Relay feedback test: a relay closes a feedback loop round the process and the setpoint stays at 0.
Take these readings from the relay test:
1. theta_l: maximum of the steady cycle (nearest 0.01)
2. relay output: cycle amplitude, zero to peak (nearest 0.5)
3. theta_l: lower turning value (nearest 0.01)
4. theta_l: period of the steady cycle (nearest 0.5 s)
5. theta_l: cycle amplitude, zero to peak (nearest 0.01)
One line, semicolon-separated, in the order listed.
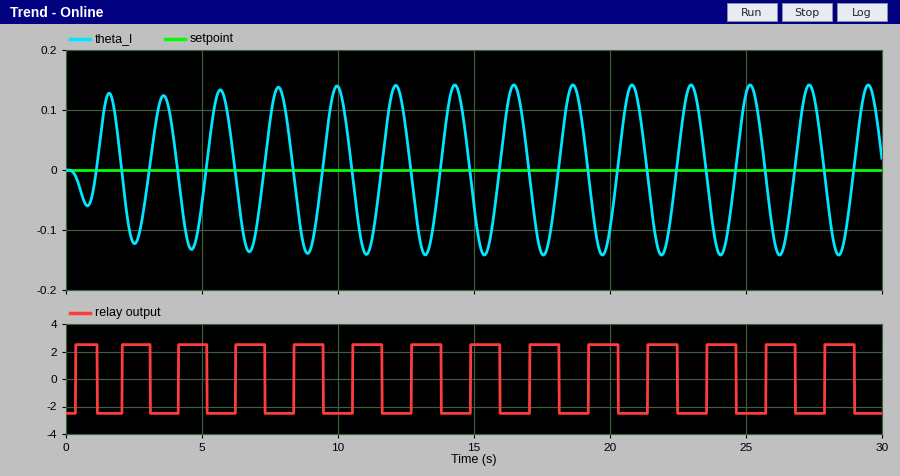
0.14; 2.5; -0.14; 2.0 s; 0.14
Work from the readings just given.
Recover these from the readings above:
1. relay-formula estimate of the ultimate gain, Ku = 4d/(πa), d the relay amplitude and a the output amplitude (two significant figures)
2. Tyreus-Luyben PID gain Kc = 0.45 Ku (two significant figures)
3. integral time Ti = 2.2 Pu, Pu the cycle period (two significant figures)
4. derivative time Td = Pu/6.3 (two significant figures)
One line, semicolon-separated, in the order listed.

23; 10; 4.4 s; 0.32 s
